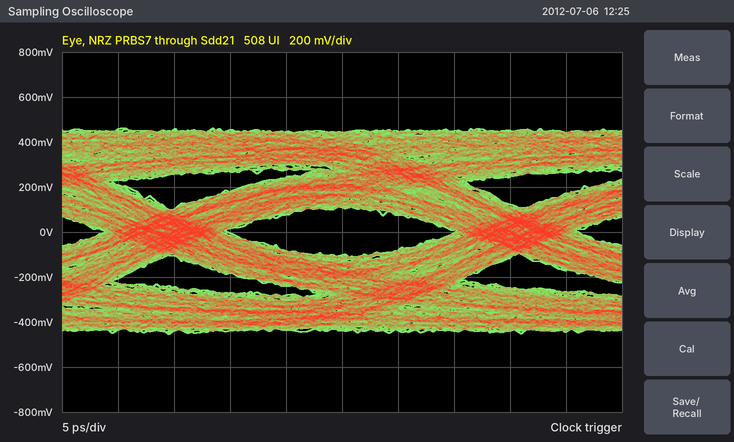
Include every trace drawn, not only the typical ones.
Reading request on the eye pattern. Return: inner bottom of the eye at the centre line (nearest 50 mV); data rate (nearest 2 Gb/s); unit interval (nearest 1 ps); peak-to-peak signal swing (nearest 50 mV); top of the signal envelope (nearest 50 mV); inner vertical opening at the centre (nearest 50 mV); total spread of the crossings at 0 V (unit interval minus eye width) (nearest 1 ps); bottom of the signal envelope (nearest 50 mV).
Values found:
-100 mV
32 Gb/s
31 ps
900 mV
450 mV
200 mV
11 ps
-450 mV
